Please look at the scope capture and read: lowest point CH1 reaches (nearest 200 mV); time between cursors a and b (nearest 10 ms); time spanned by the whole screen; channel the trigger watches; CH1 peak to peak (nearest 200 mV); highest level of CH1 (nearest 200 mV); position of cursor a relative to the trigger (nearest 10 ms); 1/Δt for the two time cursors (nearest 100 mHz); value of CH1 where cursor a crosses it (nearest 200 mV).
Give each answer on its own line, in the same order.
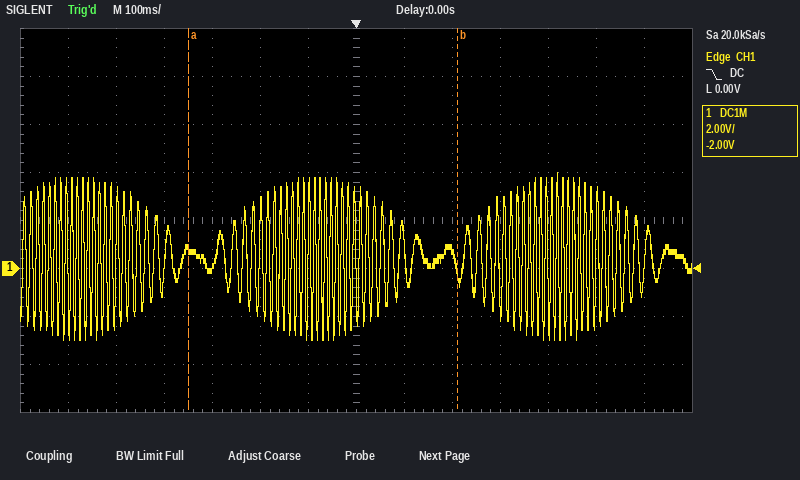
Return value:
-3.0 V
560 ms
1.4 s
CH1
7.0 V
4.0 V
-350 ms
1.8 Hz
800 mV
